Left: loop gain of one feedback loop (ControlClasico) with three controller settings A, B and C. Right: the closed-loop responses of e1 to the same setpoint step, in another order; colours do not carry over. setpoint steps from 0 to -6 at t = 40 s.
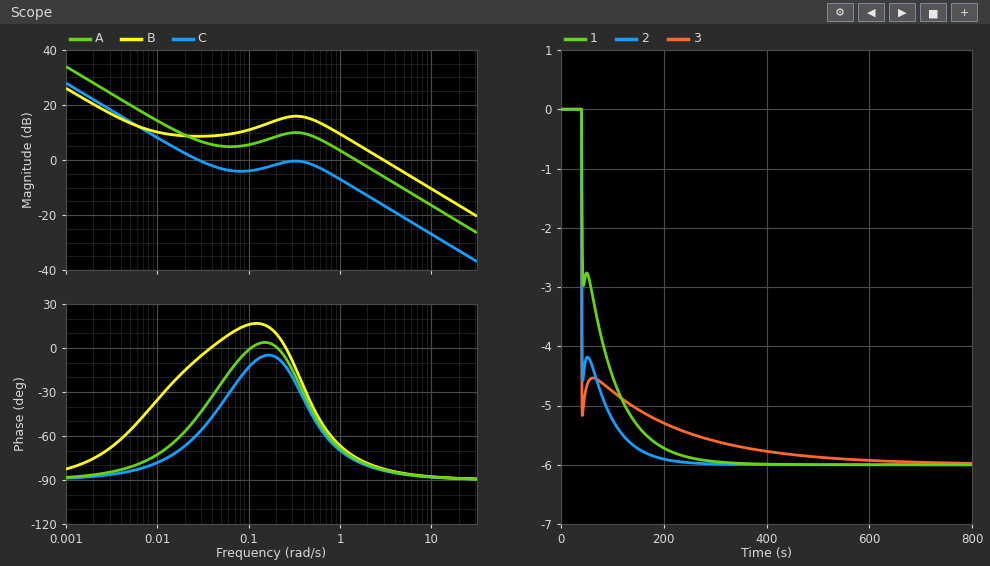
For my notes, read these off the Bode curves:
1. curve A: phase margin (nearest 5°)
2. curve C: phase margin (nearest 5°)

105°
120°
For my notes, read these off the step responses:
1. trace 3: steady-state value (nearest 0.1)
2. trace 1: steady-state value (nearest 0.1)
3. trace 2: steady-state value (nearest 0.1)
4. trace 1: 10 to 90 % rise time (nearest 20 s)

-6.0
-6.0
-6.0
120 s
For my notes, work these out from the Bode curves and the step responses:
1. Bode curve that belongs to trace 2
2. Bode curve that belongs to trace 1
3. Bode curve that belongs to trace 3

A
C
B
